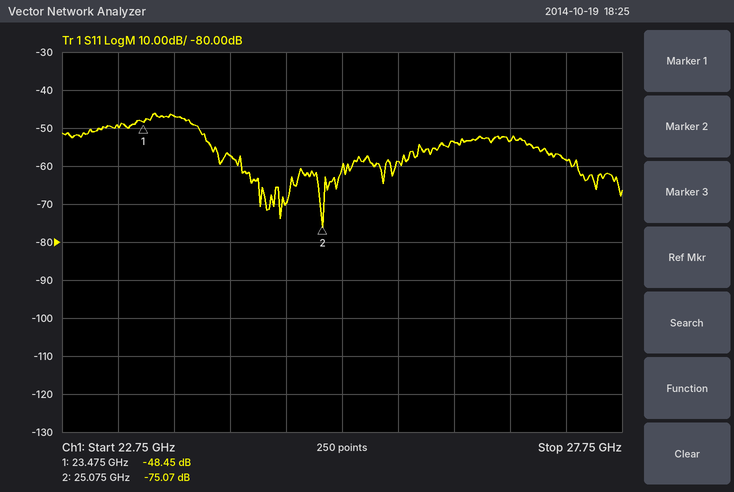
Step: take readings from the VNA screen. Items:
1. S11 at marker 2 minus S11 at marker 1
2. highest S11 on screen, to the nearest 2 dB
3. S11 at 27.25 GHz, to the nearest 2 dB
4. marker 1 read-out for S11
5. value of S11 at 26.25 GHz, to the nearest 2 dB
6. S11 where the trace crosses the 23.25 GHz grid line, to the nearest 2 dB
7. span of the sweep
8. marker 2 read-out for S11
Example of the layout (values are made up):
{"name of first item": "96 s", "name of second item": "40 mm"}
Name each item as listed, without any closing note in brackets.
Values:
{"S11 at marker 2 minus S11 at marker 1": "-26.62 dB", "highest S11 on screen, to the nearest 2 dB": "-46 dB", "S11 at 27.25 GHz, to the nearest 2 dB": "-58 dB", "marker 1 read-out for S11": "-48.45 dB", "value of S11 at 26.25 GHz, to the nearest 2 dB": "-54 dB", "S11 where the trace crosses the 23.25 GHz grid line, to the nearest 2 dB": "-50 dB", "span of the sweep": "5 GHz", "marker 2 read-out for S11": "-75.07 dB"}
